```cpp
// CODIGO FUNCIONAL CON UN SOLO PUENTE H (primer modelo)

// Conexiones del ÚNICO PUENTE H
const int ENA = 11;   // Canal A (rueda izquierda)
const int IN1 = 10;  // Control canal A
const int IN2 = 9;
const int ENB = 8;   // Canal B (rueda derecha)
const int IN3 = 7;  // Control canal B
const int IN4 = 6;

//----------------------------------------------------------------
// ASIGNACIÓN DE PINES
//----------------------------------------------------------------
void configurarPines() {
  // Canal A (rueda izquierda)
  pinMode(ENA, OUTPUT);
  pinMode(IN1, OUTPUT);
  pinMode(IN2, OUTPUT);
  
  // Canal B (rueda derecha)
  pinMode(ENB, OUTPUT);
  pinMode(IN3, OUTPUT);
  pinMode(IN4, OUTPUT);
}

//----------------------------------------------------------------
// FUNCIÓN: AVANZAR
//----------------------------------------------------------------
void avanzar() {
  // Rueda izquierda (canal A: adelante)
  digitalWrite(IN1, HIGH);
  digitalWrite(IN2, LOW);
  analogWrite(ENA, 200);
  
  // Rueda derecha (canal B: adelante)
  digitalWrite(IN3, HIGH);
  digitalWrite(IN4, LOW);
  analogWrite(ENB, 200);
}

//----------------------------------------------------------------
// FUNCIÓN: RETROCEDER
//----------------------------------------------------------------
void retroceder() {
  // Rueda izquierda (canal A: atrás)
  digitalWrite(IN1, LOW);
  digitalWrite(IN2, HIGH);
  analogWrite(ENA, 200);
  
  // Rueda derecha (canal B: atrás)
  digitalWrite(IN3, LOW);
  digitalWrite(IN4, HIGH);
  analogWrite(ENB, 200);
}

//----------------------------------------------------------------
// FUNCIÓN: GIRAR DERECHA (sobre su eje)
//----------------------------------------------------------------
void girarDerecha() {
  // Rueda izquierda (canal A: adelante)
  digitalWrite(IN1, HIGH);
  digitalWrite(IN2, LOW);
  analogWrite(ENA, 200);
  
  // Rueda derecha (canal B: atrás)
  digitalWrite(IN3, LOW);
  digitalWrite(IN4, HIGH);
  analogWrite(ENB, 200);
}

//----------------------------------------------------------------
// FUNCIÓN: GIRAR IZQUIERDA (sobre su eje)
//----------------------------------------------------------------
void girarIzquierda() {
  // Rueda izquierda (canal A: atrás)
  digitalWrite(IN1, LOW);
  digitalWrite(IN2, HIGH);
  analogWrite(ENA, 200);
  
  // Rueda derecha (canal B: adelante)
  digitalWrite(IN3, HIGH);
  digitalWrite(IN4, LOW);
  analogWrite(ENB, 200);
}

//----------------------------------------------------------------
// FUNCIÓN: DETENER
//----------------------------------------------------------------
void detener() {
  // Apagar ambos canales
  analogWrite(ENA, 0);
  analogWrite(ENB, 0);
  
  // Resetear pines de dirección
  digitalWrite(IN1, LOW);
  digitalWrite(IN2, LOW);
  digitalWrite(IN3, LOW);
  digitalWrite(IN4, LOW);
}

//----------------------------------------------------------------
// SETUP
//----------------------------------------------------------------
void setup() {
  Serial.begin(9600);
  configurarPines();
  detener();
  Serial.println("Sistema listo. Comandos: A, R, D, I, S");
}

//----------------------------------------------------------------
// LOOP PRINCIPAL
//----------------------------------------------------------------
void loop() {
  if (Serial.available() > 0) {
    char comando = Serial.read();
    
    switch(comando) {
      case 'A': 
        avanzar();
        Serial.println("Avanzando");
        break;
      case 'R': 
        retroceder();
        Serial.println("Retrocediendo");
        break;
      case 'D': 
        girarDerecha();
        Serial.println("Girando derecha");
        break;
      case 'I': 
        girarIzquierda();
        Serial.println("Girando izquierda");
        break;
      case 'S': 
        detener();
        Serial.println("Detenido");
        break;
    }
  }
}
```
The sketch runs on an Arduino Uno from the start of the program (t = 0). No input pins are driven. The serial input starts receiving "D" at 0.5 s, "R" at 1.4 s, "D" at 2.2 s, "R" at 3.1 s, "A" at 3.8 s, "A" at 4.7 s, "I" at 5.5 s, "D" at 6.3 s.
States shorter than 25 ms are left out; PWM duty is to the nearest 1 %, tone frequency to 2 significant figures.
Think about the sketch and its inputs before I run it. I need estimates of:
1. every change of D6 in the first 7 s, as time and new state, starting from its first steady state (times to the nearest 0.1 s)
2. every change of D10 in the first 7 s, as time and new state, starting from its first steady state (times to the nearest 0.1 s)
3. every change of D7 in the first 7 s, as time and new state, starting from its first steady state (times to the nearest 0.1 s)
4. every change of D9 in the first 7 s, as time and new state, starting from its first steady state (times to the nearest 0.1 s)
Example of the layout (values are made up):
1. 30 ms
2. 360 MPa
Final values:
1. 0 s low; 0.5 s high; 3.8 s low; 6.3 s high
2. 0 s low; 0.5 s high; 1.4 s low; 2.2 s high; 3.1 s low; 3.8 s high; 5.5 s low; 6.3 s high
3. 0 s low; 3.8 s high; 6.3 s low
4. 0 s low; 1.4 s high; 2.2 s low; 3.1 s high; 3.8 s low; 5.5 s high; 6.3 s low
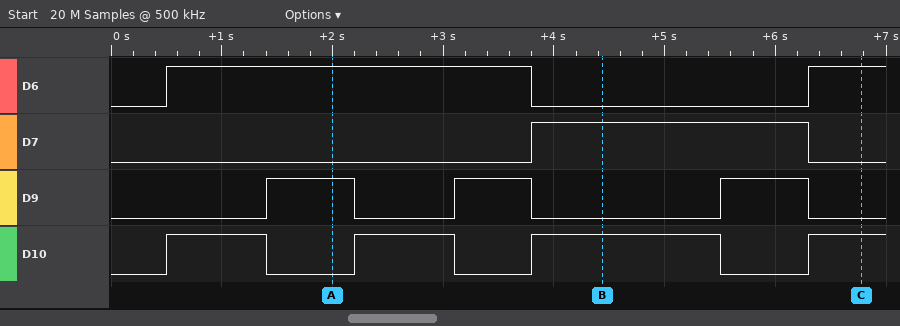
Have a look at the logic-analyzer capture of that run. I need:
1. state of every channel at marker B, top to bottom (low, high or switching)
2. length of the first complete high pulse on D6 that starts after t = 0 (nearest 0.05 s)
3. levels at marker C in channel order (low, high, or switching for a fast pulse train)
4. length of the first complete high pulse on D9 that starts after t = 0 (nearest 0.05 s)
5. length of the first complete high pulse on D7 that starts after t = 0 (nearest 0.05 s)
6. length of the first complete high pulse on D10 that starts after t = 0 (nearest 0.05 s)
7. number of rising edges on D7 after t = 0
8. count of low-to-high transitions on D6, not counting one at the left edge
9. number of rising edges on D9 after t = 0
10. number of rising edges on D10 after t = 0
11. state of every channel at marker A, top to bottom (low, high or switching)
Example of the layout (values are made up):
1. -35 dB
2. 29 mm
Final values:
1. D6 low, D7 high, D9 low, D10 high
2. 3.30 s
3. D6 high, D7 low, D9 low, D10 high
4. 0.80 s
5. 2.50 s
6. 0.90 s
7. 1
8. 2
9. 3
10. 4
11. D6 high, D7 low, D9 high, D10 low
